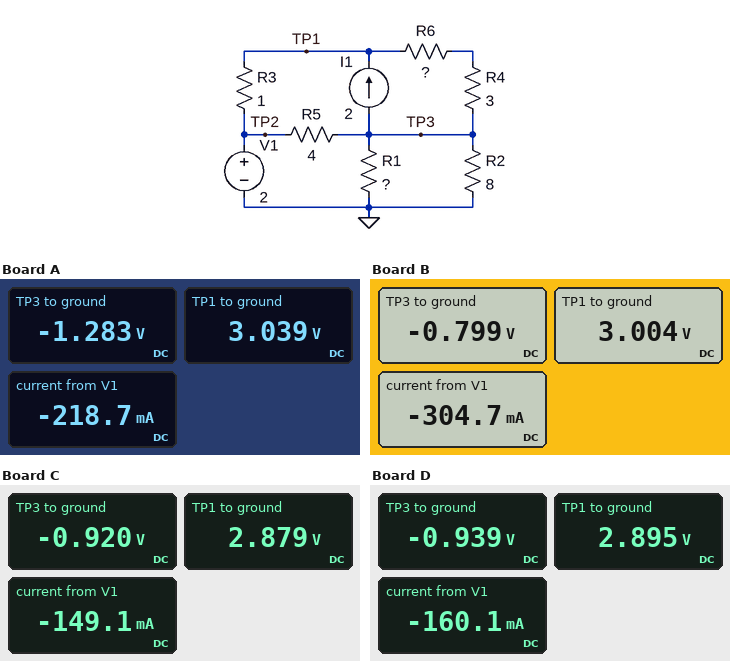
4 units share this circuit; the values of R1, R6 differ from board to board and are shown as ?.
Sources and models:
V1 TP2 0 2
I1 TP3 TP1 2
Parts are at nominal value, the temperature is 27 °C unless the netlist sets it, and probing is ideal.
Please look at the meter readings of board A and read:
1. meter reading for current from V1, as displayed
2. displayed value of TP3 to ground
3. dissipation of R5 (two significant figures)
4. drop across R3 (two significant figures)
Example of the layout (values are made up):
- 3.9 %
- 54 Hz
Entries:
- -218.7 mA
- -1.283 V
- 2.7 W
- 1.0 V
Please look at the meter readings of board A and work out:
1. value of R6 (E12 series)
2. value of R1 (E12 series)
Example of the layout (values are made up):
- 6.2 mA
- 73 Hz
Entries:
- 1.5 Ω
- 22 Ω
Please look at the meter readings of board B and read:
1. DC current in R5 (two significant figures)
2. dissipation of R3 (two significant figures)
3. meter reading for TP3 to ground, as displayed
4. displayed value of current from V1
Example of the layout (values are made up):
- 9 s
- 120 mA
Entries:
- 700 mA
- 1.0 W
- -0.799 V
- -304.7 mA
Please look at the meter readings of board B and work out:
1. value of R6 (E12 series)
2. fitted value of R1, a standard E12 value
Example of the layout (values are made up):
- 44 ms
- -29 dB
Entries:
- 0.82 Ω
- 3.9 Ω
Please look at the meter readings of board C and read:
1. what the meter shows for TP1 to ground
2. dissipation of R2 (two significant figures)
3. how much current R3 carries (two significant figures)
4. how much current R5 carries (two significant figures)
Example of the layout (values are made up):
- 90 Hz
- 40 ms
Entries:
- 2.879 V
- 110 mW
- 880 mA
- 730 mA
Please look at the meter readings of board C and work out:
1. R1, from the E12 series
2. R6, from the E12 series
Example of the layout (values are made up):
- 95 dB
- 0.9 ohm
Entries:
- 27 Ω
- 0.39 Ω
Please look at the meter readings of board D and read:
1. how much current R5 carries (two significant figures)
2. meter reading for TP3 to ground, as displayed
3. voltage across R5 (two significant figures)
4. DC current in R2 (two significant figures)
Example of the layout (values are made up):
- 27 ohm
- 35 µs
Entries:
- 730 mA
- -0.939 V
- 2.9 V
- 120 mA
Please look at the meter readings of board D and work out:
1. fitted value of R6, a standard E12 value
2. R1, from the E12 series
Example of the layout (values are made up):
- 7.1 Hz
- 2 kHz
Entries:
- 0.47 Ω
- 22 Ω
